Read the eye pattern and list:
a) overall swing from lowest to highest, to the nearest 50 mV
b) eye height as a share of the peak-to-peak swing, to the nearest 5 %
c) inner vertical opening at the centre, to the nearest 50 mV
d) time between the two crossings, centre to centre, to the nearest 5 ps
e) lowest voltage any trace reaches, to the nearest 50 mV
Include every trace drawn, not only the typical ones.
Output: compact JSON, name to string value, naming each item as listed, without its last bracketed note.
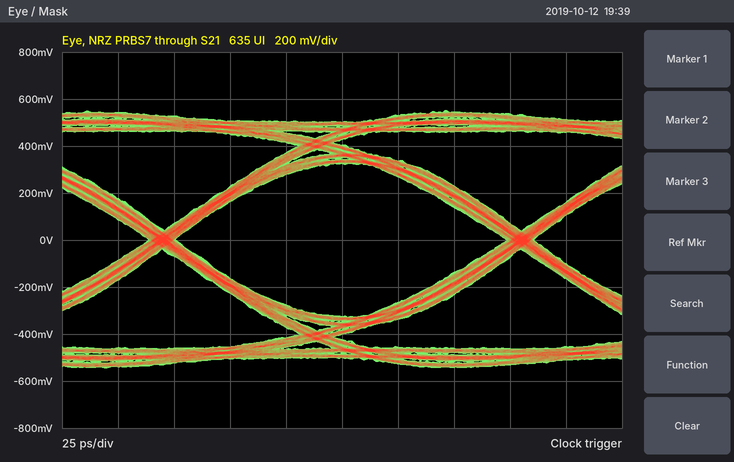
{"overall swing from lowest to highest, to the nearest 50 mV": "1.10 V", "eye height as a share of the peak-to-peak swing, to the nearest 5 %": "60 %", "inner vertical opening at the centre, to the nearest 50 mV": "650 mV", "time between the two crossings, centre to centre, to the nearest 5 ps": "160 ps", "lowest voltage any trace reaches, to the nearest 50 mV": "-550 mV"}
